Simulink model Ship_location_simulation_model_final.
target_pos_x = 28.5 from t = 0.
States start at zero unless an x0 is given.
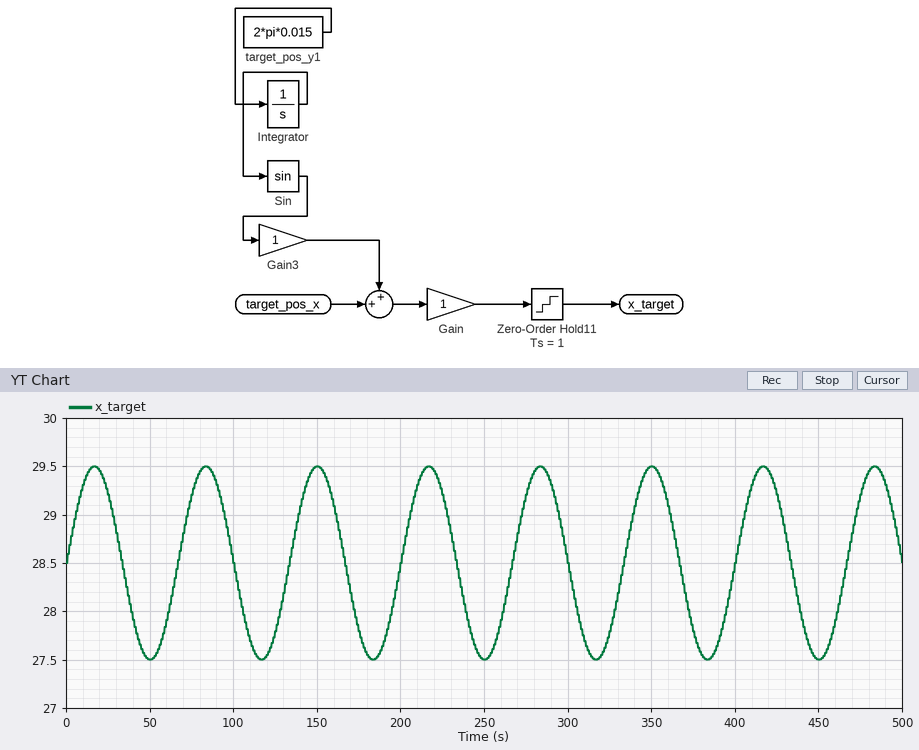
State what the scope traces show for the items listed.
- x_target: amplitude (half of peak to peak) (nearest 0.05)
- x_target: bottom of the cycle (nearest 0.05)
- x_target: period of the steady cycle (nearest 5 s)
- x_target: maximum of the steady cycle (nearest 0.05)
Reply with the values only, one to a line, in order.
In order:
1.00
27.50
65 s
29.50
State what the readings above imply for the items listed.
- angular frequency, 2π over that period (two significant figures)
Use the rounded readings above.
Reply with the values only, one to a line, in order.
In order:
0.097 rad/s
